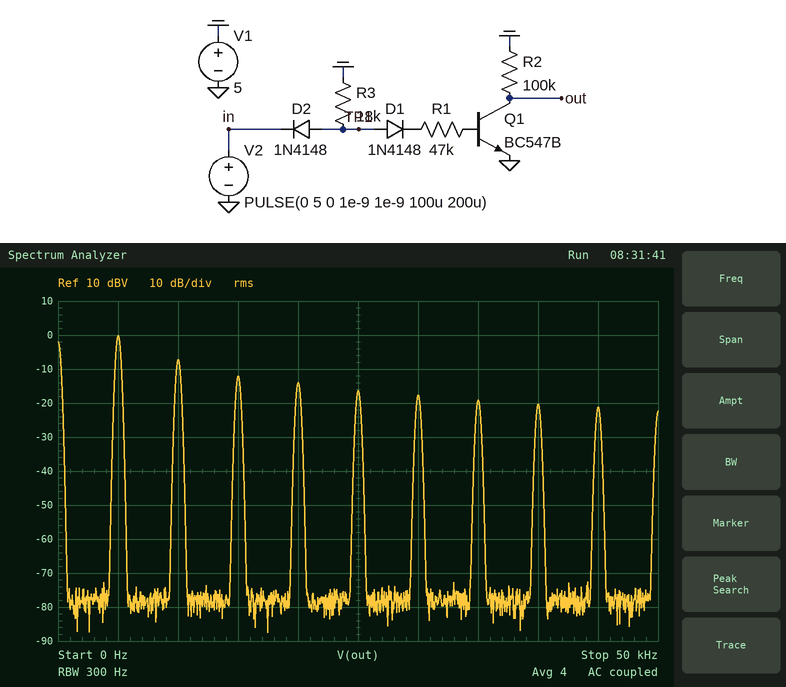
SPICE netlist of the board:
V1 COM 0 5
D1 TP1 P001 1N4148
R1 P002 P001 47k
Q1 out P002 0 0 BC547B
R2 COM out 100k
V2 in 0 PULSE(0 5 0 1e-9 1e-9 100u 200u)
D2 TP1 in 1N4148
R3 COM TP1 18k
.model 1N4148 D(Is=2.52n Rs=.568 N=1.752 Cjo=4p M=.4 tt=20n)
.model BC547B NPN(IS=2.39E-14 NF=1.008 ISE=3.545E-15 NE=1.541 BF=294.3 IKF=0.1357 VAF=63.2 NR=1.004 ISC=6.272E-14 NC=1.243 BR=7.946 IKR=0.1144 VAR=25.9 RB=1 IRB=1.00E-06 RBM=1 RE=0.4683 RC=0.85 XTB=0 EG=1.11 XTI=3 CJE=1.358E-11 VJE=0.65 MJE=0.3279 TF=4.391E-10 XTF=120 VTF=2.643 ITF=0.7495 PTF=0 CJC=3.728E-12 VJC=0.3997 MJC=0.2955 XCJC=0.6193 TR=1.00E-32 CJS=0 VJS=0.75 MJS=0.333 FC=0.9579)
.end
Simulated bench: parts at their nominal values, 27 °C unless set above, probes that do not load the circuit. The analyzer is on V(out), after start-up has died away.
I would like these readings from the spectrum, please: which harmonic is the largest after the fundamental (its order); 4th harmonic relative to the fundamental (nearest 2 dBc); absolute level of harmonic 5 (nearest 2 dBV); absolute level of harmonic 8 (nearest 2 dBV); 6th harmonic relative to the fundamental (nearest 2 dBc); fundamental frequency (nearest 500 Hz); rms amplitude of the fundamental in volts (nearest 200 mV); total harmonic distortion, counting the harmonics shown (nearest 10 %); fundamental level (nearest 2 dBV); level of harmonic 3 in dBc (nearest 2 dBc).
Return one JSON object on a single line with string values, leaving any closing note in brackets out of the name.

{"which harmonic is the largest after the fundamental": "2", "4th harmonic relative to the fundamental": "-14 dBc", "absolute level of harmonic 5": "-16 dBV", "absolute level of harmonic 8": "-20 dBV", "6th harmonic relative to the fundamental": "-18 dBc", "fundamental frequency": "5.0 kHz", "rms amplitude of the fundamental in volts": "1.0 V", "total harmonic distortion, counting the harmonics shown": "60 %", "fundamental level": "0 dBV", "level of harmonic 3 in dBc": "-12 dBc"}
